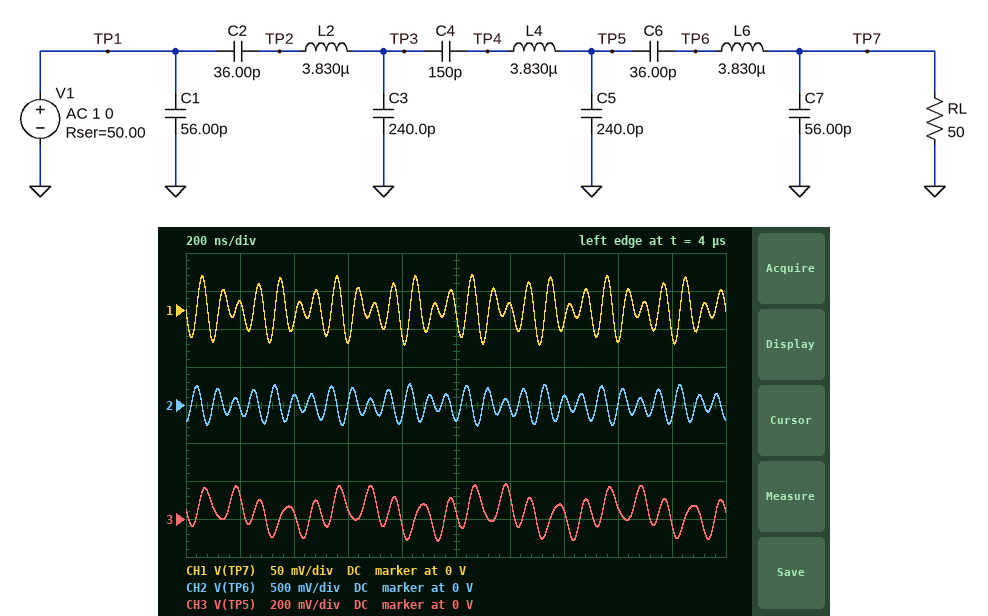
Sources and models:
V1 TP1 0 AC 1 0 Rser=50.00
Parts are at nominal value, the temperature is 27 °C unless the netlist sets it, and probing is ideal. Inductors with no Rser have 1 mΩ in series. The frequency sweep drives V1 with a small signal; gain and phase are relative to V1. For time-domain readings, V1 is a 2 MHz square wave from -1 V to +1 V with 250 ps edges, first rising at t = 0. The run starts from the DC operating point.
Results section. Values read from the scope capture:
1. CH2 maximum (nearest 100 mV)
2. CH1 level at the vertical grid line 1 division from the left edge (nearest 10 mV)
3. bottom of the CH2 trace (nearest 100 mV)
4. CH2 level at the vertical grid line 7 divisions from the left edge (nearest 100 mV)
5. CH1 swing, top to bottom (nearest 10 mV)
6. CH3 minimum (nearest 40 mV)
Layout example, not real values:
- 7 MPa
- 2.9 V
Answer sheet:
- 300 mV
- 10 mV
- -300 mV
- 100 mV
- 90 mV
- -120 mV
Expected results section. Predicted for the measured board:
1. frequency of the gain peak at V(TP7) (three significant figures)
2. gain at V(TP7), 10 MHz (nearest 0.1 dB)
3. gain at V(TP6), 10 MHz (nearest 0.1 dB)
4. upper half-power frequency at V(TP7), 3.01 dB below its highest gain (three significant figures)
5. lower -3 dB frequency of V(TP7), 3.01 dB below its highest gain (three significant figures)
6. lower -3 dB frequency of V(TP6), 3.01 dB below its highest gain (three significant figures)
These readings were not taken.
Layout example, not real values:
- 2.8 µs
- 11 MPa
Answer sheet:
- 9.35 MHz
- -21.8 dB
- -8.1 dB
- 9.44 MHz
- 9.27 MHz
- 9.27 MHz
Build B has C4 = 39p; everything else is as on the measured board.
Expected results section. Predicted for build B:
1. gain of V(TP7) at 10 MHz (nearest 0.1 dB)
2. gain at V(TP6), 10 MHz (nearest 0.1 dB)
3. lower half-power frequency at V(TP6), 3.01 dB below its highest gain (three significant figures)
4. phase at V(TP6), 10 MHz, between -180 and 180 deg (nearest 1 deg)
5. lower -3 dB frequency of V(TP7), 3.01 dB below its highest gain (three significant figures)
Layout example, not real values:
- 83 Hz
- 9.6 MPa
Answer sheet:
- -39.9 dB
- -26.3 dB
- 13.5 MHz
- 137 deg
- 13.4 MHz
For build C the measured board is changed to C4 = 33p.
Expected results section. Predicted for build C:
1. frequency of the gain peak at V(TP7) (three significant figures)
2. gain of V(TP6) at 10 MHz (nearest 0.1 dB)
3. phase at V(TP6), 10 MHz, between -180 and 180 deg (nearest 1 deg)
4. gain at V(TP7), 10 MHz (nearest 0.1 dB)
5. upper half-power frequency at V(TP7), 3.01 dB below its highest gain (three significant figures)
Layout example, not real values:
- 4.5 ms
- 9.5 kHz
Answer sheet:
- 16.6 MHz
- -28.4 dB
- 137 deg
- -42.1 dB
- 16.9 MHz
